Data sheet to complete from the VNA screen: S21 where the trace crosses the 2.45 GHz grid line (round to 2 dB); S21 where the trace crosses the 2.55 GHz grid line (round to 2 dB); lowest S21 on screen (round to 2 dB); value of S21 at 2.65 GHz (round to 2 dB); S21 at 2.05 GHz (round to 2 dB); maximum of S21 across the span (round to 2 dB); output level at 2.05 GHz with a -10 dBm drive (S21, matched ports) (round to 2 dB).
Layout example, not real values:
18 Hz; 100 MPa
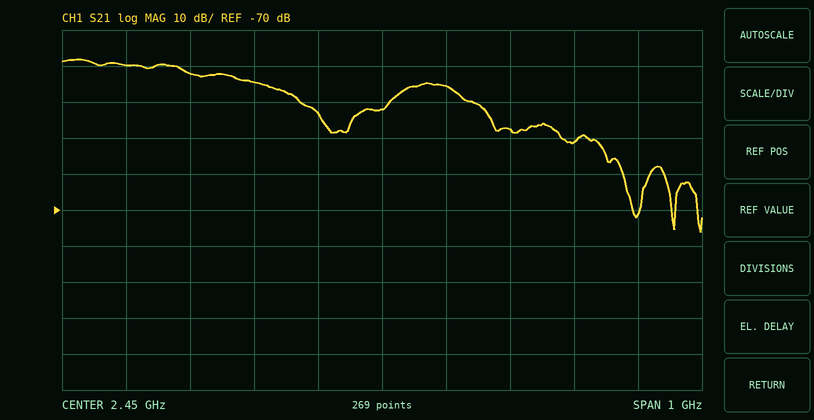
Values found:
-42 dB; -36 dB; -76 dB; -48 dB; -30 dB; -28 dB; -40 dBm
